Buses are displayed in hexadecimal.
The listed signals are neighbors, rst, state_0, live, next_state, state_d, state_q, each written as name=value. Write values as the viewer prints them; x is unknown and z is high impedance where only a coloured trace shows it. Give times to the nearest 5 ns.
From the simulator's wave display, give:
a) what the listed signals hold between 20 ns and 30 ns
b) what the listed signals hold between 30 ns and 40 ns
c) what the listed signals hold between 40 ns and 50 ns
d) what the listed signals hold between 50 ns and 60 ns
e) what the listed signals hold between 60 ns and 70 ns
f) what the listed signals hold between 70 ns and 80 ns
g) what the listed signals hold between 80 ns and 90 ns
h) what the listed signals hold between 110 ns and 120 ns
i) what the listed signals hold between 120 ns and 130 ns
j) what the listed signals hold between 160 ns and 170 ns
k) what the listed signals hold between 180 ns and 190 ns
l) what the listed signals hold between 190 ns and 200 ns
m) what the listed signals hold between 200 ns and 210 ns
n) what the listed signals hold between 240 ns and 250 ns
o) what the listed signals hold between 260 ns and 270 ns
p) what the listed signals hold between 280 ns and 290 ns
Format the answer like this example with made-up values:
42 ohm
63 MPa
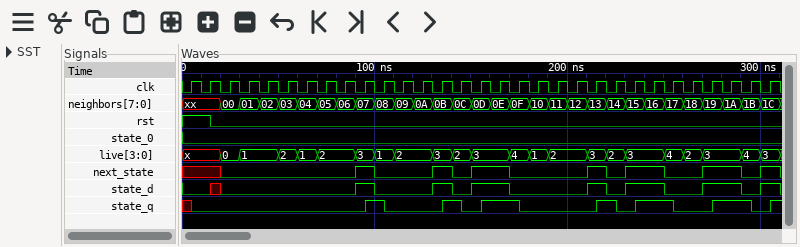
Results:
neighbors=00, rst=0, state_0=0, live=0, next_state=0, state_d=0, state_q=0
neighbors=01, rst=0, state_0=0, live=1, next_state=0, state_d=0, state_q=0
neighbors=02, rst=0, state_0=0, live=1, next_state=0, state_d=0, state_q=0
neighbors=03, rst=0, state_0=0, live=2, next_state=0, state_d=0, state_q=0
neighbors=04, rst=0, state_0=0, live=1, next_state=0, state_d=0, state_q=0
neighbors=05, rst=0, state_0=0, live=2, next_state=0, state_d=0, state_q=0
neighbors=06, rst=0, state_0=0, live=2, next_state=0, state_d=0, state_q=0
neighbors=09, rst=0, state_0=0, live=2, next_state=0, state_d=0, state_q=0
neighbors=0A, rst=0, state_0=0, live=2, next_state=0, state_d=0, state_q=0
neighbors=0E, rst=0, state_0=0, live=3, next_state=1, state_d=1, state_q=1
neighbors=10, rst=0, state_0=0, live=1, next_state=0, state_d=0, state_q=0
neighbors=11, rst=0, state_0=0, live=2, next_state=0, state_d=0, state_q=0
neighbors=12, rst=0, state_0=0, live=2, next_state=0, state_d=0, state_q=0
neighbors=16, rst=0, state_0=0, live=3, next_state=1, state_d=1, state_q=1
neighbors=18, rst=0, state_0=0, live=2, next_state=0, state_d=0, state_q=0
neighbors=1A, rst=0, state_0=0, live=3, next_state=1, state_d=1, state_q=1
